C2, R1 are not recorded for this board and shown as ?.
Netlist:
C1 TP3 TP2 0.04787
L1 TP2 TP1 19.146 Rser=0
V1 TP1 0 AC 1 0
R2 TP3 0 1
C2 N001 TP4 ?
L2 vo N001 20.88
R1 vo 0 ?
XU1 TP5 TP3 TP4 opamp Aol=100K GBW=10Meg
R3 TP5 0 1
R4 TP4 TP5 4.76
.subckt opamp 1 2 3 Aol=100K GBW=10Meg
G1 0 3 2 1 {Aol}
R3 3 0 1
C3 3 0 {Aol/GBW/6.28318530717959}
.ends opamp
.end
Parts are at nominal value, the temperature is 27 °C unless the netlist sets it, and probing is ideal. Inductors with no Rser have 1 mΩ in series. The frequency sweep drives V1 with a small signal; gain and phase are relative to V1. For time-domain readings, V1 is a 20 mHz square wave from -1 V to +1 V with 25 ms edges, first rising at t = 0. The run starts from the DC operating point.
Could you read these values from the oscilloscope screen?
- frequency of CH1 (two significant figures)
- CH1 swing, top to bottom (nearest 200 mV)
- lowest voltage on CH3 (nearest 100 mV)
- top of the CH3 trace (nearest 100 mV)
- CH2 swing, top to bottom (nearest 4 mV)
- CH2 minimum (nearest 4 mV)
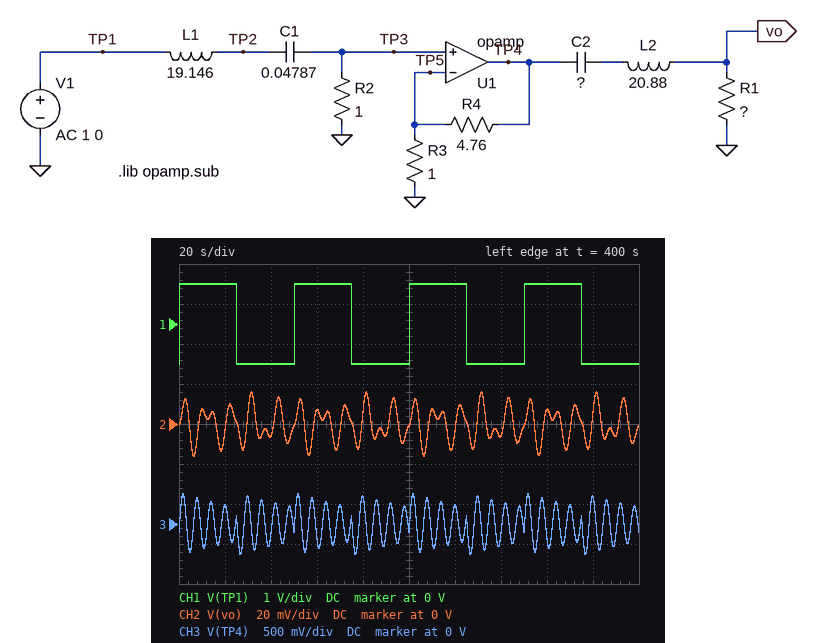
20 mHz
2.0 V
-400 mV
400 mV
32 mV
-16 mV
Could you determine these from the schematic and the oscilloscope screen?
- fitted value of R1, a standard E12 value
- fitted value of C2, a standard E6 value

0.33 Ω
150 mF
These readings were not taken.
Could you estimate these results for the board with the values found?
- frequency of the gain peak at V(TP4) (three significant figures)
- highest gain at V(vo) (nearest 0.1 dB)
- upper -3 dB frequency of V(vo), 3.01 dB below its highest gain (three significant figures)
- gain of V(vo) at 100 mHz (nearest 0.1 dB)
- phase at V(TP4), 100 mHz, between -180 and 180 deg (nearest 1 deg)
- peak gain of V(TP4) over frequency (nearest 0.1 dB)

166 mHz
-13.2 dB
91.3 mHz
-29.0 dB
87 deg
15.2 dB
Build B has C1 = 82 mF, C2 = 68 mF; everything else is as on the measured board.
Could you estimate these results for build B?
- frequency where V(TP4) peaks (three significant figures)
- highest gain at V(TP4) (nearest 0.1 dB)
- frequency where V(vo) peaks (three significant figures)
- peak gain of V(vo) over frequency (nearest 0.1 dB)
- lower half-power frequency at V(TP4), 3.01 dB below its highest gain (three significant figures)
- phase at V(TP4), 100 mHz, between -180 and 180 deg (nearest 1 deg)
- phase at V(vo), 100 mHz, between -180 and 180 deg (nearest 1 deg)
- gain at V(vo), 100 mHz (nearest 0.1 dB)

127 mHz
15.2 dB
133 mHz
10.0 dB
123 mHz
82 deg
170 deg
-32.1 dB
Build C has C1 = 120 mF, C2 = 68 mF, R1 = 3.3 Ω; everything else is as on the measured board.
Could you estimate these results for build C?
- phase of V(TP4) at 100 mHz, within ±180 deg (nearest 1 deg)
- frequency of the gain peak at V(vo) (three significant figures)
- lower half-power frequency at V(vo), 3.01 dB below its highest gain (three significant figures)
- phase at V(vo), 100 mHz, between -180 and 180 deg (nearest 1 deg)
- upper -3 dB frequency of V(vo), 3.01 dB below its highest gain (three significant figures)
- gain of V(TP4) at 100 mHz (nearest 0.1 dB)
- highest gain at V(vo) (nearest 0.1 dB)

51 deg
106 mHz
102 mHz
123 deg
111 mHz
11.2 dB
6.5 dB
